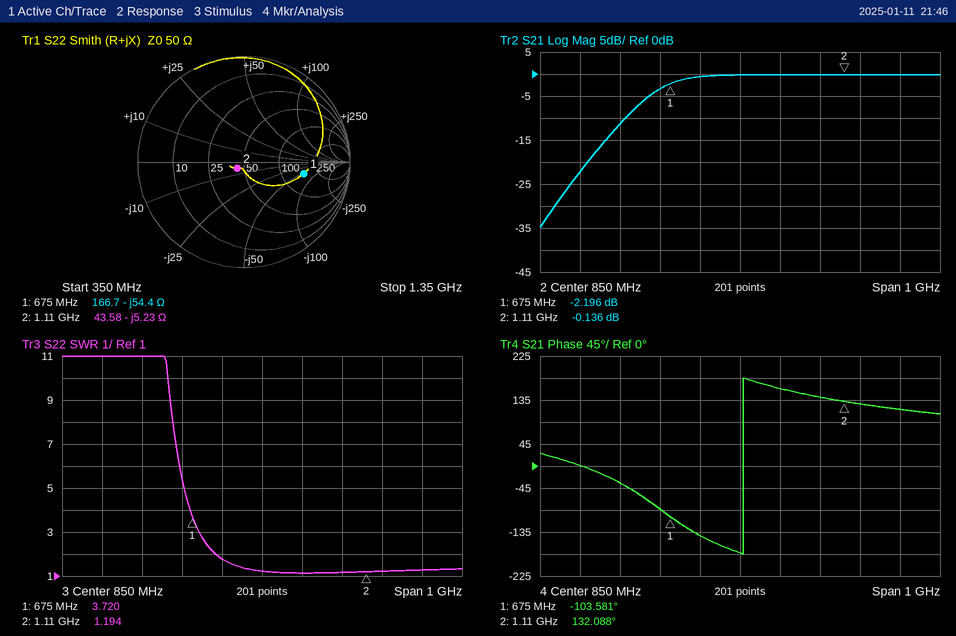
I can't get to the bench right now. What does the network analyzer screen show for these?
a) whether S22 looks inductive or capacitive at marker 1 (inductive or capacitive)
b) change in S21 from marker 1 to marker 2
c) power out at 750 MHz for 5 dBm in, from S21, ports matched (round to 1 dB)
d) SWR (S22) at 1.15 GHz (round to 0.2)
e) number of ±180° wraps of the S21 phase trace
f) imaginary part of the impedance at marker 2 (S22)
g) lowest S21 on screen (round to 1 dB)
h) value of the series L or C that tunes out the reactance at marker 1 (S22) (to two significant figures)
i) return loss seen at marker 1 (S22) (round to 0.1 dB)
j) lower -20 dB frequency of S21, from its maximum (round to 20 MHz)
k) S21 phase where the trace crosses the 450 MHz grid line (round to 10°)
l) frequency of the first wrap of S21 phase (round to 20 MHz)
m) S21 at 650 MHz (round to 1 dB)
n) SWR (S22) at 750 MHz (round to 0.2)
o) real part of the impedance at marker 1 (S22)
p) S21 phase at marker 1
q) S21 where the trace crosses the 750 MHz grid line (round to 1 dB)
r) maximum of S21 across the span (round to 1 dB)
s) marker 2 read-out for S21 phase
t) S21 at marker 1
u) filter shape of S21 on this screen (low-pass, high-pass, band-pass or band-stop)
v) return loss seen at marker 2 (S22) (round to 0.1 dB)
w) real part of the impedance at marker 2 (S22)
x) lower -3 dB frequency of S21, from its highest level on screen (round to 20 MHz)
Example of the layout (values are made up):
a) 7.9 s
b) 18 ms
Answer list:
a) capacitive
b) 2.060 dB
c) 4 dBm
d) 1.2
e) 1
f) -5.23 Ω
g) -35 dB
h) 13 nH
i) 4.8 dB
j) 460 MHz
k) 0°
l) 860 MHz
m) -3 dB
n) 1.8
o) 166.7 Ω
p) -103.581°
q) -1 dB
r) 0 dB
s) 132.088°
t) -2.196 dB
u) high-pass
v) 21.1 dB
w) 43.58 Ω
x) 660 MHz
